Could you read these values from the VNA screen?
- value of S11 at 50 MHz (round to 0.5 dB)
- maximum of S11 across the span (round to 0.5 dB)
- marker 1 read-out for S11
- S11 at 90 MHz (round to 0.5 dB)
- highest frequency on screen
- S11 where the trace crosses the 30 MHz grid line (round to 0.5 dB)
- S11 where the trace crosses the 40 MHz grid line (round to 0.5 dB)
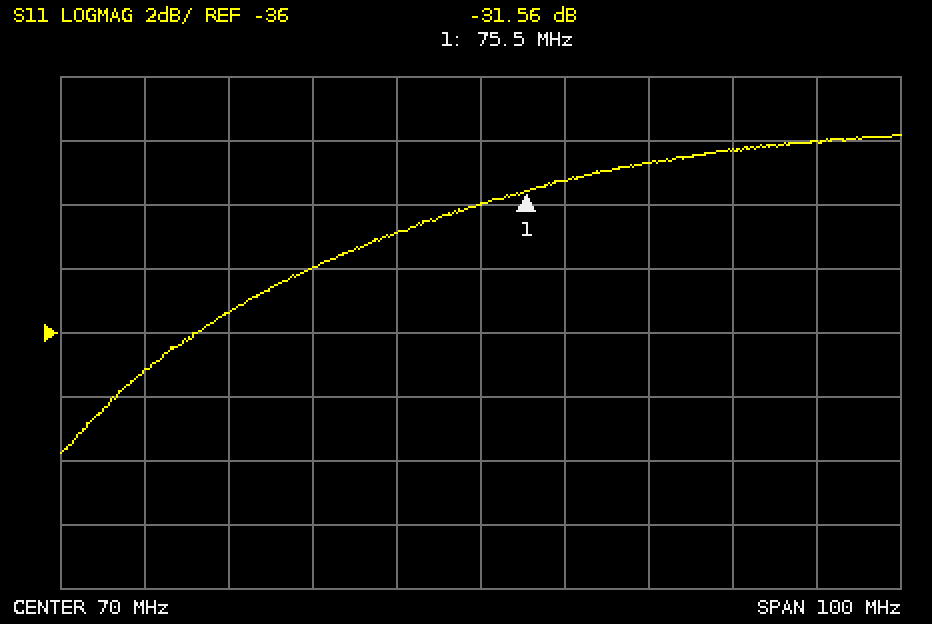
-34.0 dB
-30.0 dB
-31.56 dB
-30.5 dB
120 MHz
-37.0 dB
-35.5 dB
